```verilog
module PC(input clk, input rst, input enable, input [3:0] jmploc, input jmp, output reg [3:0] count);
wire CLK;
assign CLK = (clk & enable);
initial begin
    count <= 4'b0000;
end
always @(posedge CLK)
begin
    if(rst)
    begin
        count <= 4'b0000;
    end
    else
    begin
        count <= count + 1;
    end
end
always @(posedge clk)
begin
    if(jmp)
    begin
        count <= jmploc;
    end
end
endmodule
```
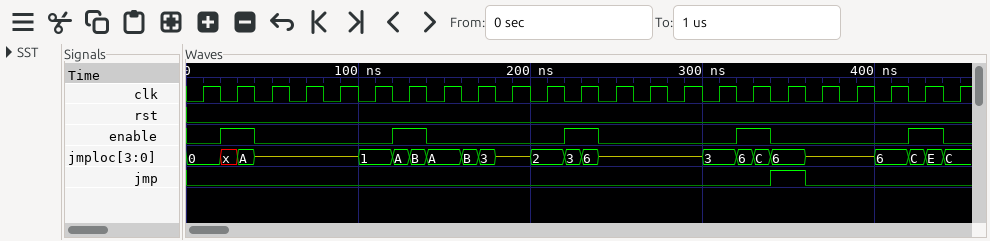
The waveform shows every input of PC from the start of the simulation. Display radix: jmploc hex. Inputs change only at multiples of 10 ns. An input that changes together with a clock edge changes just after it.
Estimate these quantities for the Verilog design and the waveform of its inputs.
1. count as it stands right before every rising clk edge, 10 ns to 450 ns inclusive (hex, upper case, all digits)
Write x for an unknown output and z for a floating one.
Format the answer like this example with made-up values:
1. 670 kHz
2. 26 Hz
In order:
1. 0, 0, 1, 1, 1, 1, 1, 2, 2, 2, 2, 2, 3, 3, 3, 3, 3, 4, 6, 6, 6, 6, 7
